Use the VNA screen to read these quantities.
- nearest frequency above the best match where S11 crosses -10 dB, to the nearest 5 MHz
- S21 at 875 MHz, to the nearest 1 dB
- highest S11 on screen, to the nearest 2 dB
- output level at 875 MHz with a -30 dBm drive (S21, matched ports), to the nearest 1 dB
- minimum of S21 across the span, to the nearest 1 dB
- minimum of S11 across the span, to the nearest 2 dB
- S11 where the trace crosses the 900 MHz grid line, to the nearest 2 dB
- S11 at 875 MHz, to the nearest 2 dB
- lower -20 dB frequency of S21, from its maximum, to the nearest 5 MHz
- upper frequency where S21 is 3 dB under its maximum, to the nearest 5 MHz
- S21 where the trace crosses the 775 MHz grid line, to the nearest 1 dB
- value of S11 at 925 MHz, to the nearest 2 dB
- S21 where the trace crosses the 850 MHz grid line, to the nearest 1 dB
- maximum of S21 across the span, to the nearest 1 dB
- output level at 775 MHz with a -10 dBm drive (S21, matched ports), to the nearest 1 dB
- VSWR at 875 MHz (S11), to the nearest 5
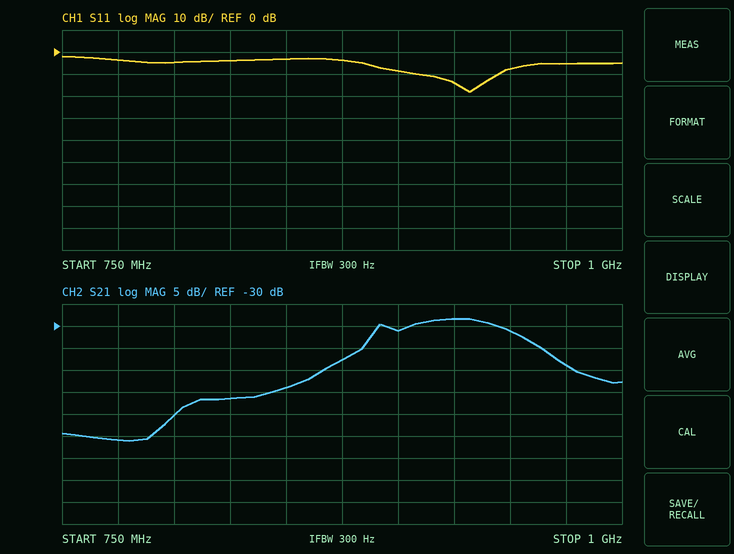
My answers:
945 MHz
-38 dB
-2 dB
-68 dBm
-56 dB
-18 dB
-8 dB
-4 dB
805 MHz
950 MHz
-56 dB
-14 dB
-44 dB
-28 dB
-66 dBm
5
